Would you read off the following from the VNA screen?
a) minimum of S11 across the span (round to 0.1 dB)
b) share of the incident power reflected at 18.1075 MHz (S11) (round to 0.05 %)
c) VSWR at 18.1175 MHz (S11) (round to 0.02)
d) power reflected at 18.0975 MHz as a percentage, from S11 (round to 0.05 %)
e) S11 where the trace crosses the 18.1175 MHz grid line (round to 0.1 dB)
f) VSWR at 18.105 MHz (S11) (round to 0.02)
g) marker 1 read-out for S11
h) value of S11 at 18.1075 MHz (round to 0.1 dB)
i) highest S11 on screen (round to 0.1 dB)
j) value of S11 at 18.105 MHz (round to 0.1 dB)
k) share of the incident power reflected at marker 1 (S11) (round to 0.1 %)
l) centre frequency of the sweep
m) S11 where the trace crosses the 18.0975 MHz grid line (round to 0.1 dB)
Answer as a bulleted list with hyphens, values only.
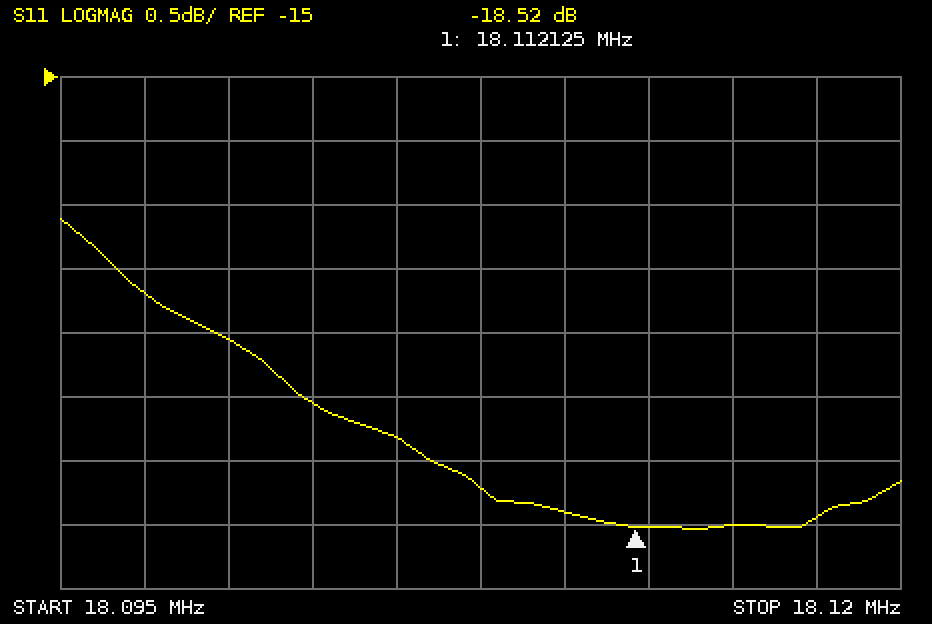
- -18.5 dB
- 1.50 %
- 1.28
- 2.15 %
- -18.4 dB
- 1.30
- -18.52 dB
- -18.2 dB
- -16.1 dB
- -17.8 dB
- 1.4 %
- 18.1075 MHz
- -16.7 dB
